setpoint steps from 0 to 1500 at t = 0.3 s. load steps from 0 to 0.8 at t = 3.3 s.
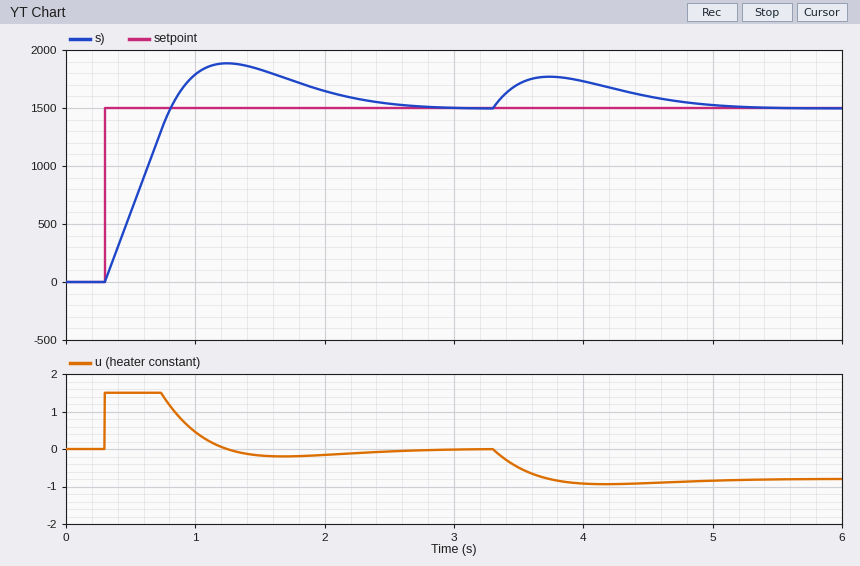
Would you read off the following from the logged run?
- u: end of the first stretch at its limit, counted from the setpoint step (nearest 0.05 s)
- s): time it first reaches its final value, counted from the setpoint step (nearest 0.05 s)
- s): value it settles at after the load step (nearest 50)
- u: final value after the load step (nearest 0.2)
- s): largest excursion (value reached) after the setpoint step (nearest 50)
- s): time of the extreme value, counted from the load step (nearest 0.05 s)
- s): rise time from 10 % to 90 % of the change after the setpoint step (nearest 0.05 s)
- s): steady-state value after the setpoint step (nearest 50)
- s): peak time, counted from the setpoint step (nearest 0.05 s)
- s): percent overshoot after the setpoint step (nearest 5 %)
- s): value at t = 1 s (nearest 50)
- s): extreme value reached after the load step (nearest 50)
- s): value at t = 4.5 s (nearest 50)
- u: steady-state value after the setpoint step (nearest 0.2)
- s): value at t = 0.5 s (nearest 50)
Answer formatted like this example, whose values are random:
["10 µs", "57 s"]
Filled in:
["0.45 s", "0.50 s", "1500", "-0.8", "1900", "0.45 s", "0.40 s", "1500", "0.95 s", "25 %", "1800", "1750", "1600", "0.0", "600"]
